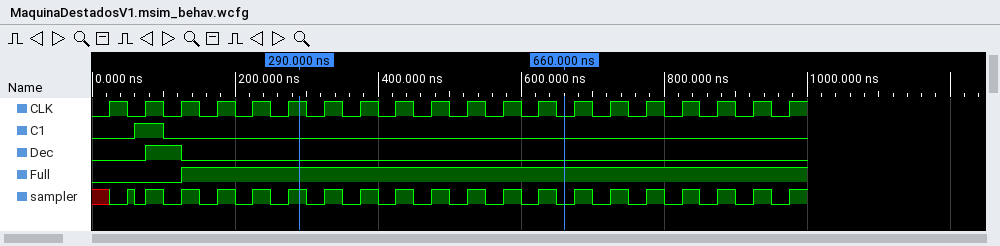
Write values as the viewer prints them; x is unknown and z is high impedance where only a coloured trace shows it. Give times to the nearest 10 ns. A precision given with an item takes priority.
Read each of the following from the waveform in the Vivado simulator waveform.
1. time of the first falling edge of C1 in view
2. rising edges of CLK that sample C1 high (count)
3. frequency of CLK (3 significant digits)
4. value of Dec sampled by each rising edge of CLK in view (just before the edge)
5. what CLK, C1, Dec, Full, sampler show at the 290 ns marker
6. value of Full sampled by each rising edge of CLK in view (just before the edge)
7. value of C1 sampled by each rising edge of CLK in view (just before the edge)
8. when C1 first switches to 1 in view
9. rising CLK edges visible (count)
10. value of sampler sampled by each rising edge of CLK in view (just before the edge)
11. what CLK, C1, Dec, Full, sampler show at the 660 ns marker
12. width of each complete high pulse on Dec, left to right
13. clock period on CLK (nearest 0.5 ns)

100 ns
1
20.0 MHz
0 0 1 0 0 0 0 0 0 0 0 0 0 0 0 0 0 0 0 0
CLK=1, C1=0, Dec=0, Full=1, sampler=1
0 0 0 1 1 1 1 1 1 1 1 1 1 1 1 1 1 1 1 1
0 1 0 0 0 0 0 0 0 0 0 0 0 0 0 0 0 0 0 0
60 ns
20
x 0 0 0 0 0 0 0 0 0 0 0 0 0 0 0 0 0 0 0
CLK=0, C1=0, Dec=0, Full=1, sampler=0
50 ns
50 ns
